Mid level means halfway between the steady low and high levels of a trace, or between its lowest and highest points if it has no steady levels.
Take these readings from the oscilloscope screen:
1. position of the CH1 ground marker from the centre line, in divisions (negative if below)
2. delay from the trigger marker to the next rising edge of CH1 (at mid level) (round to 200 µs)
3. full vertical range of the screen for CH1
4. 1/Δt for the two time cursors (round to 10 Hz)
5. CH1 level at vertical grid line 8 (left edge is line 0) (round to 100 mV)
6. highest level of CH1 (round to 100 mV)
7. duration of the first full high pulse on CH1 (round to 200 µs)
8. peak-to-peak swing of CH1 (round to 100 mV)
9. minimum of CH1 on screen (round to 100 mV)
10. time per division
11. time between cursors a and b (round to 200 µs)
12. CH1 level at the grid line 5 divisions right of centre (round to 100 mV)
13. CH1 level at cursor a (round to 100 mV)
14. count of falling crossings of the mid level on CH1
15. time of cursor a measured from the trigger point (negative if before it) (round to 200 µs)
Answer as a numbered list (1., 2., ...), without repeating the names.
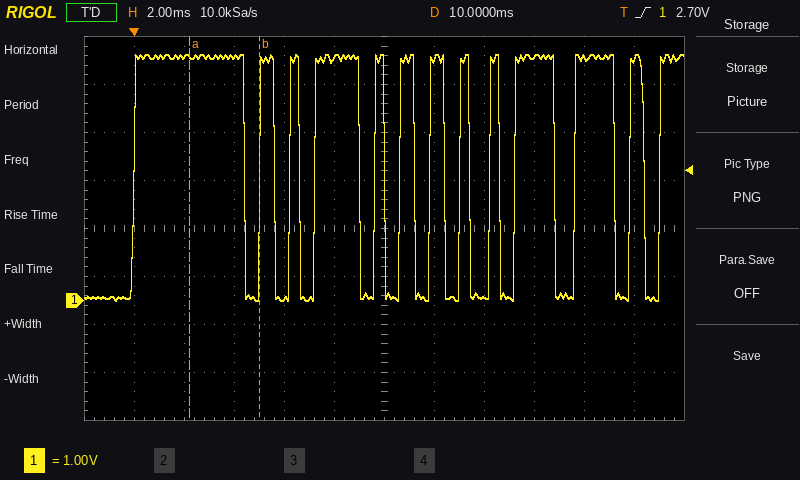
1. -1.5 div
2. 5.0 ms
3. 8 V
4. 360 Hz
5. 100 mV
6. 5.1 V
7. 4.4 ms
8. 5.1 V
9. 0.0 V
10. 2 ms
11. 2.8 ms
12. 5.0 V
13. 5.1 V
14. 12
15. +2.2 ms
